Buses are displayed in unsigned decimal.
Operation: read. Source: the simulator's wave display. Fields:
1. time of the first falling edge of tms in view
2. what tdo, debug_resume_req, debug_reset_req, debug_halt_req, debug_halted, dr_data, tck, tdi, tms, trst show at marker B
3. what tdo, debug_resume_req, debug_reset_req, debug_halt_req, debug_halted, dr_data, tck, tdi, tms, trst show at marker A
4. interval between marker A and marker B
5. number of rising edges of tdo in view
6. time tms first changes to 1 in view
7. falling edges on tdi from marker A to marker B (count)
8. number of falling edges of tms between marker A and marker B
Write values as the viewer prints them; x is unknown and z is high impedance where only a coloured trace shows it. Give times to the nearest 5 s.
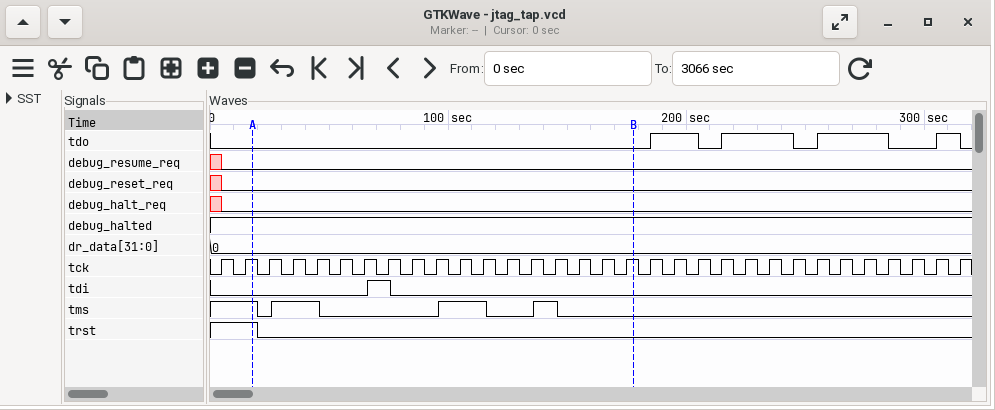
20 s
tdo=0, debug_resume_req=0, debug_reset_req=0, debug_halt_req=0, debug_halted=1, dr_data=0, tck=1, tdi=0, tms=0, trst=0
tdo=0, debug_resume_req=0, debug_reset_req=0, debug_halt_req=0, debug_halted=1, dr_data=0, tck=1, tdi=0, tms=1, trst=1
160 s
4
25 s
1
4
